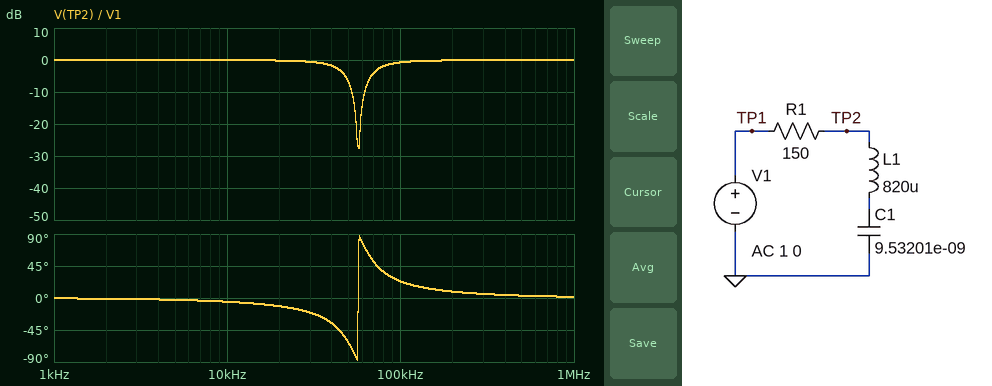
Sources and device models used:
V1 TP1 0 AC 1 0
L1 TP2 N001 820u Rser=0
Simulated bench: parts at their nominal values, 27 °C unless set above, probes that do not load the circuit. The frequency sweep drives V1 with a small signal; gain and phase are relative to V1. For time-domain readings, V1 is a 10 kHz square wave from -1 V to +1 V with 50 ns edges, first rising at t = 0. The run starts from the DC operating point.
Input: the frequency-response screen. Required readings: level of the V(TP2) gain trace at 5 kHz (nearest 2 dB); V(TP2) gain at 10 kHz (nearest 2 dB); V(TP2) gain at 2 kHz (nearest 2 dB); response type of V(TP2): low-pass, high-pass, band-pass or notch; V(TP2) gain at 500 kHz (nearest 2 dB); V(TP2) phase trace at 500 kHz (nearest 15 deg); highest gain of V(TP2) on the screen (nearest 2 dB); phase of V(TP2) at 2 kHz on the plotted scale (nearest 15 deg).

0 dB
0 dB
0 dB
notch
0 dB
0 deg
0 dB
0 deg
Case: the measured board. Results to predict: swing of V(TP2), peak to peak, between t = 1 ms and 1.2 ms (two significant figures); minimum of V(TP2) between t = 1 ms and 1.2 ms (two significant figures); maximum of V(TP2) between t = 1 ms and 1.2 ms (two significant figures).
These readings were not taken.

2.6 V
-1.3 V
1.3 V
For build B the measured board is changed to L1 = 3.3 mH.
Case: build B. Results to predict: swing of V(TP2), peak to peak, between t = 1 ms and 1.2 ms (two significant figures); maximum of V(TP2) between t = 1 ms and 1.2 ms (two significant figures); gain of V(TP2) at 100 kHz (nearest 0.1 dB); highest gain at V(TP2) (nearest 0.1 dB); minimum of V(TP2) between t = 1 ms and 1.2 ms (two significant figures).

2.7 V
1.4 V
0 dB
0 dB
-1.4 V
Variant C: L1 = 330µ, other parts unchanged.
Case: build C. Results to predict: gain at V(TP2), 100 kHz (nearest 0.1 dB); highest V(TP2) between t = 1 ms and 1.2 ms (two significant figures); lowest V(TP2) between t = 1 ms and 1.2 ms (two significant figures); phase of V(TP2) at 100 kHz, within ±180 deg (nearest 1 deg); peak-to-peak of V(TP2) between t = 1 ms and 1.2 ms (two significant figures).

-11.7 dB
1.2 V
-1.2 V
75 deg
2.5 V
